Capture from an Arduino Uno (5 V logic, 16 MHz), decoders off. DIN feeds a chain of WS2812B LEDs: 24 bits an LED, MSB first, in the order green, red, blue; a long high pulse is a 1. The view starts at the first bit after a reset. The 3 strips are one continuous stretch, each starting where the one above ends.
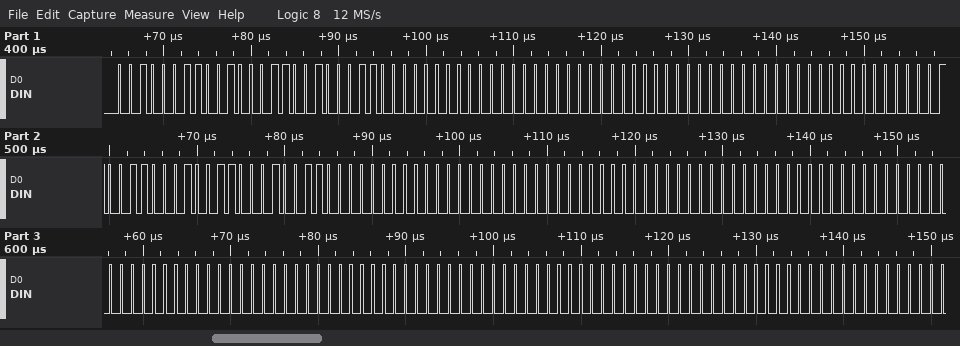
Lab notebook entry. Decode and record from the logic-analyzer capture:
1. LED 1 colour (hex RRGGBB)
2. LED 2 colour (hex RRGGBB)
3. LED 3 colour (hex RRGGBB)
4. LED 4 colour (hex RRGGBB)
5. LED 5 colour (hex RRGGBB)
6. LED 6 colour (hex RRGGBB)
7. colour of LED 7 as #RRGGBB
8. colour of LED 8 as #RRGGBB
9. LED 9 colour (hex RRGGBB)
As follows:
#232323
#000000
#000000
#131313
#000000
#000000
#000000
#000000
#000000
